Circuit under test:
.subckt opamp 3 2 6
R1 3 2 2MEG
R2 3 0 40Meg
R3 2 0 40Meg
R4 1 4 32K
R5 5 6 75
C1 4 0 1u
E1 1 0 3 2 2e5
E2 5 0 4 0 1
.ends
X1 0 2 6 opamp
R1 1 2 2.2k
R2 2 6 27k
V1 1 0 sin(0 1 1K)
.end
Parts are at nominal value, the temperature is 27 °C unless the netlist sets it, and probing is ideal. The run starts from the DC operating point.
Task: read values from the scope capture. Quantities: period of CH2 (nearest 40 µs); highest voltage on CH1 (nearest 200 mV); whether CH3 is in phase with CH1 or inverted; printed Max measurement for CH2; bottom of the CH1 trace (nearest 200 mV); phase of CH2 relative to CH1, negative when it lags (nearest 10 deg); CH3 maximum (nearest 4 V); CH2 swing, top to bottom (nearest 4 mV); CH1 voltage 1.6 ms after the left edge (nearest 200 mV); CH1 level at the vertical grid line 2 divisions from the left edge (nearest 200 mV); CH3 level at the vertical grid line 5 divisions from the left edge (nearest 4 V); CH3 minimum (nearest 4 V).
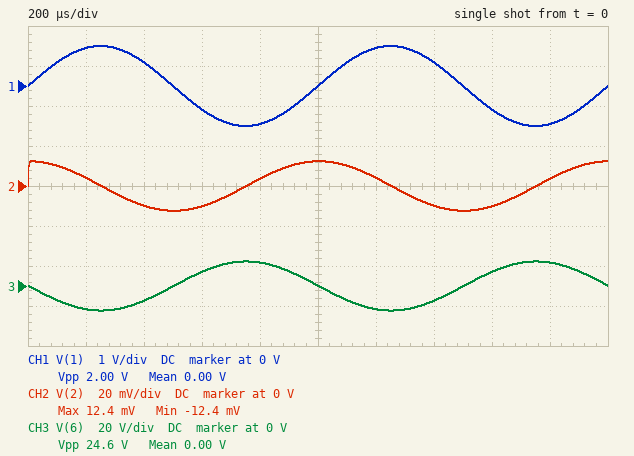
1.00 ms
1.0 V
inverted
12.4 mV
-1.0 V
90 deg
12 V
24 mV
-600 mV
600 mV
0 V
-12 V
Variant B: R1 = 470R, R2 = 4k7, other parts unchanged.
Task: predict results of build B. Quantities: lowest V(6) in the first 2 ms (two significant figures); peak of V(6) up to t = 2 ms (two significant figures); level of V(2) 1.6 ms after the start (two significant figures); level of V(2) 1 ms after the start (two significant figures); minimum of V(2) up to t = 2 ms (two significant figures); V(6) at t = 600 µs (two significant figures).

-10 V
10 V
-8.4 mV
10 mV
-10 mV
5.8 V
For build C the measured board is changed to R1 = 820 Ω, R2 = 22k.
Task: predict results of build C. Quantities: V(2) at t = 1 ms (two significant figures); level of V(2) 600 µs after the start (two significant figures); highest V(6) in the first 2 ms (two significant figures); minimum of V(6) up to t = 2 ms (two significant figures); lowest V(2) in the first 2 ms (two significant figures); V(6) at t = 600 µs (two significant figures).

27 mV
-22 mV
27 V
-27 V
-27 mV
15 V
